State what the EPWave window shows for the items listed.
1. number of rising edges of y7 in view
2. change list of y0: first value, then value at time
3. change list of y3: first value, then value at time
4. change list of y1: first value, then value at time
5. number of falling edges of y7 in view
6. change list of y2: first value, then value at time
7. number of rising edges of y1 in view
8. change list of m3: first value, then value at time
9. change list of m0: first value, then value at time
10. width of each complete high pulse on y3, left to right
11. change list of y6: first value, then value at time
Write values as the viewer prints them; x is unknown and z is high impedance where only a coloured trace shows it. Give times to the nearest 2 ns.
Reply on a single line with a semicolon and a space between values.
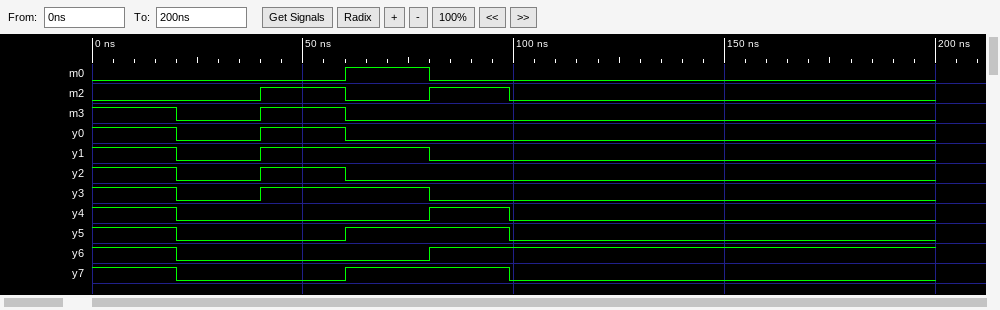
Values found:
1; 1, 0 at 20 ns, 1 at 40 ns, 0 at 60 ns; 1, 0 at 20 ns, 1 at 40 ns, 0 at 80 ns; 1, 0 at 20 ns, 1 at 40 ns, 0 at 80 ns; 2; 1, 0 at 20 ns, 1 at 40 ns, 0 at 60 ns; 1; 1, 0 at 20 ns, 1 at 40 ns, 0 at 60 ns; 0, 1 at 60 ns, 0 at 80 ns; 40 ns; 1, 0 at 20 ns, 1 at 80 ns
